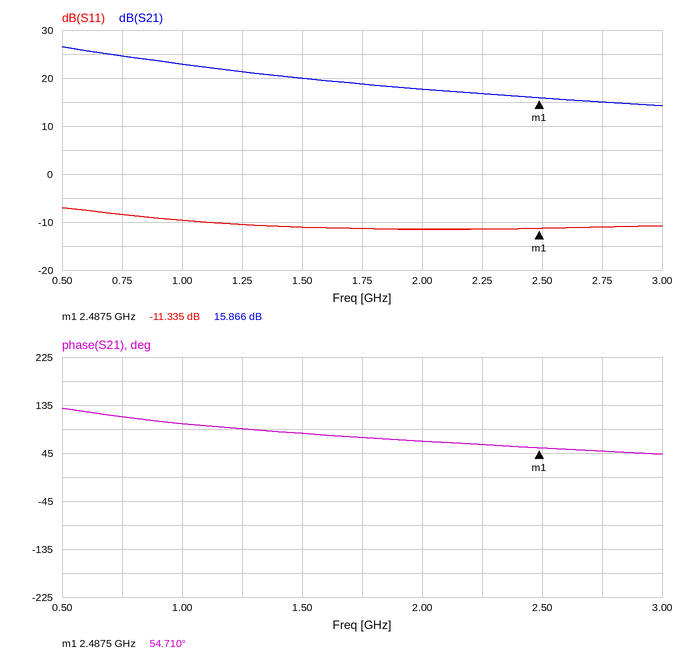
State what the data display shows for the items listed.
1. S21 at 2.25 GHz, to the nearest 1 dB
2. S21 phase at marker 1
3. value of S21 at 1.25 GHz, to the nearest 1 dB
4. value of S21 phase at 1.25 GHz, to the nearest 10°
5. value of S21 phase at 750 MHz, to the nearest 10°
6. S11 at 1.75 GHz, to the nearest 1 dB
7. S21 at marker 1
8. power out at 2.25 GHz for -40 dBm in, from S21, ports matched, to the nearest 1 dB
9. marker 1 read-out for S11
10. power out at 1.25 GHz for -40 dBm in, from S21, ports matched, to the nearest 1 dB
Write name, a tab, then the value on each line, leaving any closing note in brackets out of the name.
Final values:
S21 at 2.25 GHz, to the nearest 1 dB	17 dB
S21 phase at marker 1	54.710°
value of S21 at 1.25 GHz, to the nearest 1 dB	21 dB
value of S21 phase at 1.25 GHz, to the nearest 10°	90°
value of S21 phase at 750 MHz, to the nearest 10°	110°
S11 at 1.75 GHz, to the nearest 1 dB	-11 dB
S21 at marker 1	15.866 dB
power out at 2.25 GHz for -40 dBm in, from S21, ports matched, to the nearest 1 dB	-23 dBm
marker 1 read-out for S11	-11.335 dB
power out at 1.25 GHz for -40 dBm in, from S21, ports matched, to the nearest 1 dB	-19 dBm
